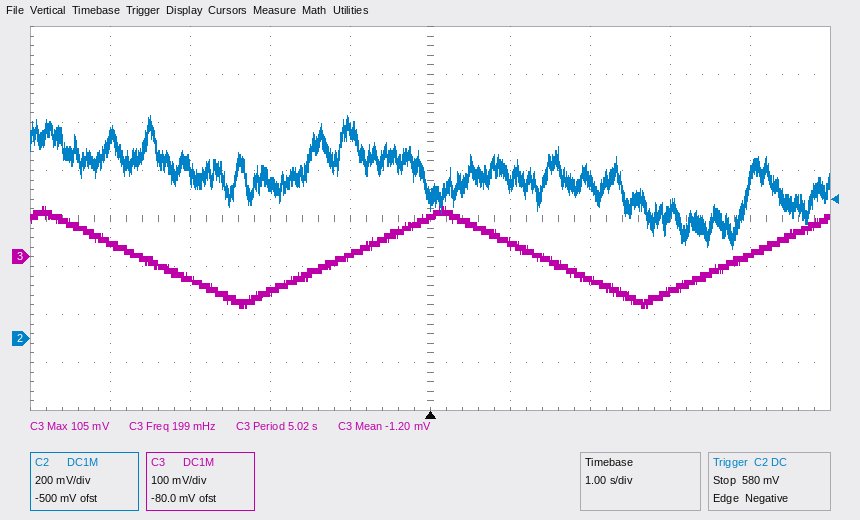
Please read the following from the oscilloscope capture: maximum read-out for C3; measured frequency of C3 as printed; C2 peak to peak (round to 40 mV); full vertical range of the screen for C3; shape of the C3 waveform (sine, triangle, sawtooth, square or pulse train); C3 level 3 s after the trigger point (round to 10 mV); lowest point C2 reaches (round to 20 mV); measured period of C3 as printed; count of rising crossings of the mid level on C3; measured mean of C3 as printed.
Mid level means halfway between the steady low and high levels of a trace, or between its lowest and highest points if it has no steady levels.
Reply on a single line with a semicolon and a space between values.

105 mV; 199 mHz; 560 mV; 800 mV; triangle; -70 mV; 380 mV; 5.02 s; 2; -1.20 mV
